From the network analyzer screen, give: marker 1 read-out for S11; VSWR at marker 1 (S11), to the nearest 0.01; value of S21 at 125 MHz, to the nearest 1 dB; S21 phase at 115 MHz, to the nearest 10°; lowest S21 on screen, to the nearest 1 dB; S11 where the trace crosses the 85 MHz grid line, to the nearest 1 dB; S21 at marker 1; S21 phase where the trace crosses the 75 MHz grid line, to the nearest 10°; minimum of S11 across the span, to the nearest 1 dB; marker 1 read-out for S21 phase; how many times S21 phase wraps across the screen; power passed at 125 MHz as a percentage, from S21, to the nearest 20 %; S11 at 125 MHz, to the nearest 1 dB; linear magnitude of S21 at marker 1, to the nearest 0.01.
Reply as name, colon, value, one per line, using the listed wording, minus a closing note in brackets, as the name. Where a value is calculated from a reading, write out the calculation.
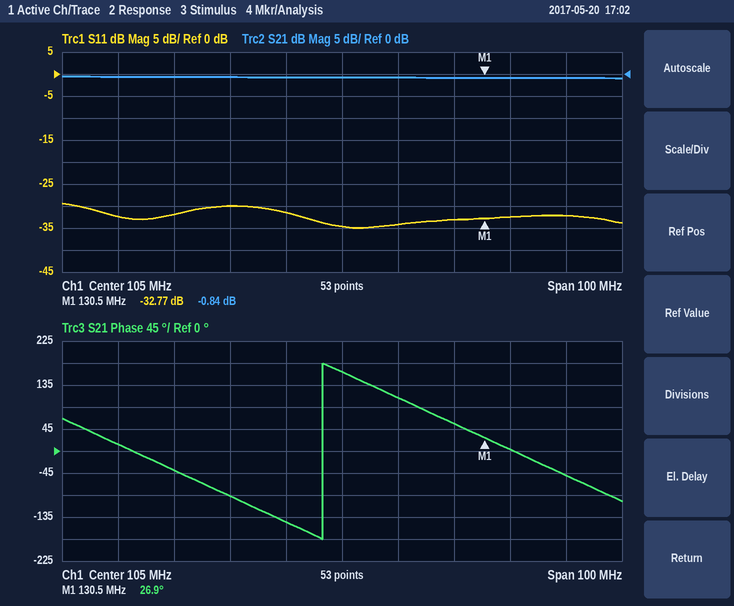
marker 1 read-out for S11: -32.77 dB
VSWR at marker 1 (S11), to the nearest 0.01: (1 + 0.0230)/(1 − 0.0230) ≈ 1.05
value of S21 at 125 MHz, to the nearest 1 dB: -1 dB
S21 phase at 115 MHz, to the nearest 10°: 110°
lowest S21 on screen, to the nearest 1 dB: -1 dB
S11 where the trace crosses the 85 MHz grid line, to the nearest 1 dB: -30 dB
S21 at marker 1: -0.84 dB
S21 phase where the trace crosses the 75 MHz grid line, to the nearest 10°: -40°
minimum of S11 across the span, to the nearest 1 dB: -35 dB
marker 1 read-out for S21 phase: 26.9°
how many times S21 phase wraps across the screen: 1
power passed at 125 MHz as a percentage, from S21, to the nearest 20 %: 10^(-1/10) ≈ 79.4 %, so 80 % to the nearest 20 %
S11 at 125 MHz, to the nearest 1 dB: -33 dB
linear magnitude of S21 at marker 1, to the nearest 0.01: 10^(-0.84/20) ≈ 0.91
